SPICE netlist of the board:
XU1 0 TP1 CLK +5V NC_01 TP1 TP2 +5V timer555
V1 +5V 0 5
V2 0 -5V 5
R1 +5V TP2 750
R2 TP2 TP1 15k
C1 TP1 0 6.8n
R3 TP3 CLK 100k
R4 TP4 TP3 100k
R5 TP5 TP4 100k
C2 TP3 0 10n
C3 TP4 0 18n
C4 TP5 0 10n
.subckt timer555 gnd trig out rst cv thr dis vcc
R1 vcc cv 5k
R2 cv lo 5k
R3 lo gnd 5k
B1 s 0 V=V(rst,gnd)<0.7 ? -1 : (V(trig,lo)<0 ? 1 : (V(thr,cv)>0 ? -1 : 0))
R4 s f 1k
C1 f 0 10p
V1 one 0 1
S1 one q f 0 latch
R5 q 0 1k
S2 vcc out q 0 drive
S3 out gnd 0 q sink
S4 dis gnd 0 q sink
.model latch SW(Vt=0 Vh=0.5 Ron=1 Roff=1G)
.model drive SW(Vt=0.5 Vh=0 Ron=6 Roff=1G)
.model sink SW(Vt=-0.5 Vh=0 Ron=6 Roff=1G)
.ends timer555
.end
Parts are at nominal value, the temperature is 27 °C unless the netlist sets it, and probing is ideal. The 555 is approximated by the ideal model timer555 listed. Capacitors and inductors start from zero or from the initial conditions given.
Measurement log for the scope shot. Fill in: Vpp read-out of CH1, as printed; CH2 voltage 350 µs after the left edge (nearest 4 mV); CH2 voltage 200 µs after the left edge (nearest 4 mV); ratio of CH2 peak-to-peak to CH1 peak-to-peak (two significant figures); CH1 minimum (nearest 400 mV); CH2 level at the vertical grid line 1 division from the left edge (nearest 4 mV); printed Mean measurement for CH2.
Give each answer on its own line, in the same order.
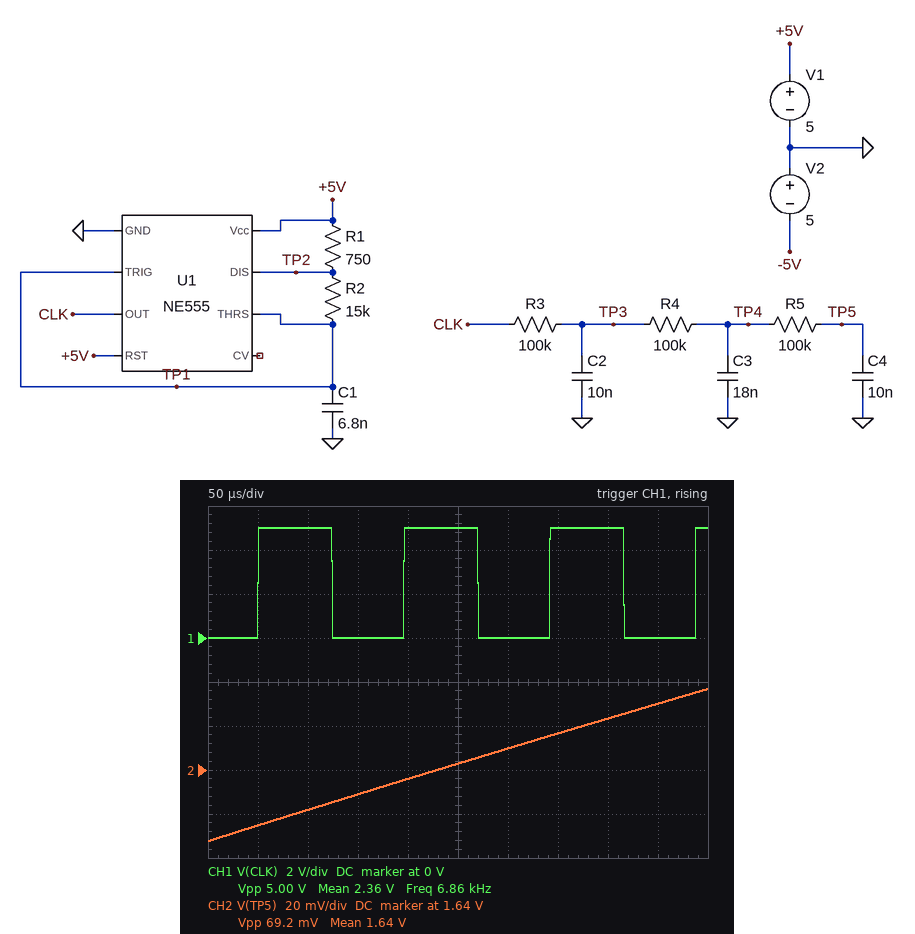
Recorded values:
5.00 V
1.656 V
1.636 V
0.014
0 V
1.616 V
1.64 V
